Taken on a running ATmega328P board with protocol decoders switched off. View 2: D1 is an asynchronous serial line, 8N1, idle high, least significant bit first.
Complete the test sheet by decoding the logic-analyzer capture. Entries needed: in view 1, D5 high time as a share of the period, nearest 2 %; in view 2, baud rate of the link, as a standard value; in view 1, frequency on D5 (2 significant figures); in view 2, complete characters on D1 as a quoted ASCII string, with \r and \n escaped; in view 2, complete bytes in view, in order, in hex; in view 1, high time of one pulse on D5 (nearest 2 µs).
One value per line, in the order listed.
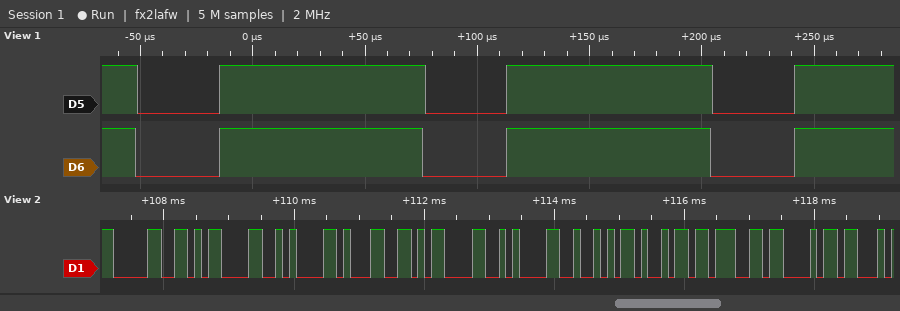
72 %
9600 baud
7.8 kHz
"0\r\n1\r\nRigh"
30 0D 0A 31 0D 0A 52 69 67 68
92 µs
